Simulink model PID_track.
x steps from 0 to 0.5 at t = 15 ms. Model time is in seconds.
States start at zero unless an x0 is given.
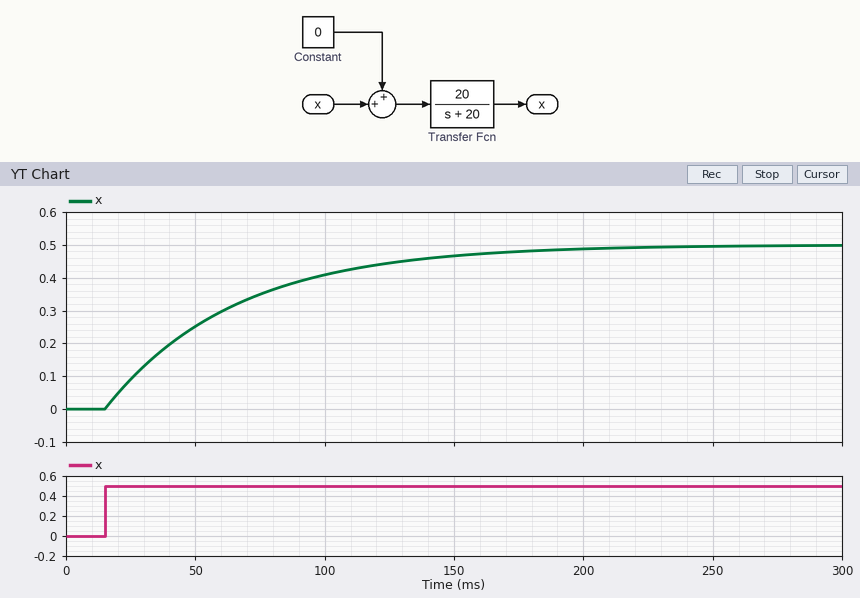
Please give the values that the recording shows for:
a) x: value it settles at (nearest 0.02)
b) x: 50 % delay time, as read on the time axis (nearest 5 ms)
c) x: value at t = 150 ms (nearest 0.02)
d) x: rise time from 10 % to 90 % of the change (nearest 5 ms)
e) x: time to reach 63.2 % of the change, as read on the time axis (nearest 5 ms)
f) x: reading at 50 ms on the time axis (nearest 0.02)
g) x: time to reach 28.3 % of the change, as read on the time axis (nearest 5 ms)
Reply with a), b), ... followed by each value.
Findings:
a) 0.50
b) 50 ms
c) 0.46
d) 110 ms
e) 65 ms
f) 0.26
g) 30 ms
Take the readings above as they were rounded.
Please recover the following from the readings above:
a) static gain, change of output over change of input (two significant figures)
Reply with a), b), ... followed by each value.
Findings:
a) 1.0
